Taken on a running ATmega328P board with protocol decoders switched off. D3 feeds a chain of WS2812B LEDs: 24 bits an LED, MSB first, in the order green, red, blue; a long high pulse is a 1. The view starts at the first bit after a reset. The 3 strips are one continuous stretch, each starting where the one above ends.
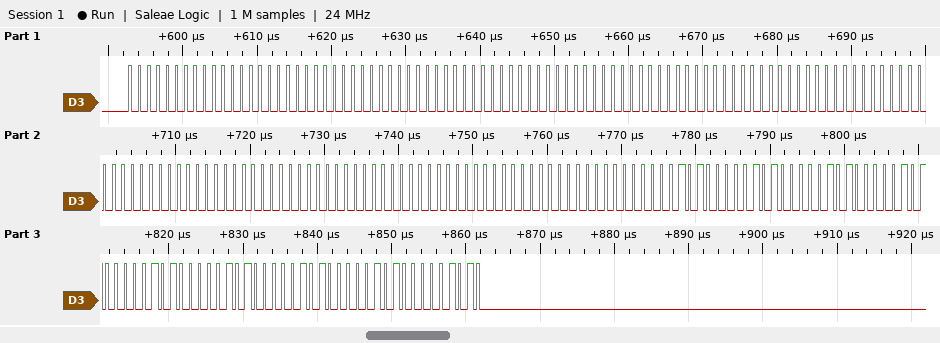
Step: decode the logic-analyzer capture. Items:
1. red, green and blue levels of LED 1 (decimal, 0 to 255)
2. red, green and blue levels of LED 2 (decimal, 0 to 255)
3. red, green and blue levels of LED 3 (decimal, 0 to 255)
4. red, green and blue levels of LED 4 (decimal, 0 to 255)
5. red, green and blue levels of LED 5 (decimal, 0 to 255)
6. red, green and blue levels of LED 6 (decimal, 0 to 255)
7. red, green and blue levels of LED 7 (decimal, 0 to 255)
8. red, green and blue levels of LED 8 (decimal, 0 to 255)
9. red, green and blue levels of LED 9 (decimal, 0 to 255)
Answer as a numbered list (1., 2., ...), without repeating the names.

1. 0, 0, 0
2. 0, 0, 0
3. 0, 0, 0
4. 0, 0, 0
5. 0, 0, 0
6. 0, 0, 0
7. 10, 10, 10
8. 10, 10, 10
9. 10, 10, 10
